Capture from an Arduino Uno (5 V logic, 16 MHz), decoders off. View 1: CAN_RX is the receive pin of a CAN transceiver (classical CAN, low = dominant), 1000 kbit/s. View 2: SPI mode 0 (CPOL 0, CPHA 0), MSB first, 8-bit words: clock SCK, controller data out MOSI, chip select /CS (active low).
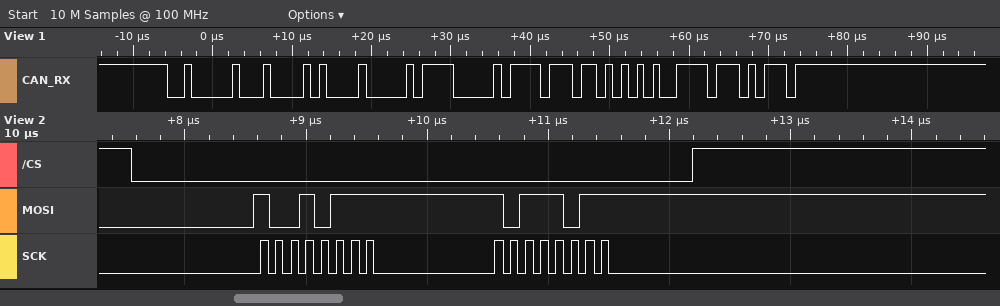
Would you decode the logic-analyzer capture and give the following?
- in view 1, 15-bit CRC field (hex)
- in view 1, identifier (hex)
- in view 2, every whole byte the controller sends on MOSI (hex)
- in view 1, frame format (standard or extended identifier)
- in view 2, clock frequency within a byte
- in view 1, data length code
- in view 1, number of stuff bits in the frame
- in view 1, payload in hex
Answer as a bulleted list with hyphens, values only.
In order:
- 0x1EEB
- 0x201
- 97 BB
- standard
- 8 MHz
- 5
- 3
- 08 1E 07 BB 55
